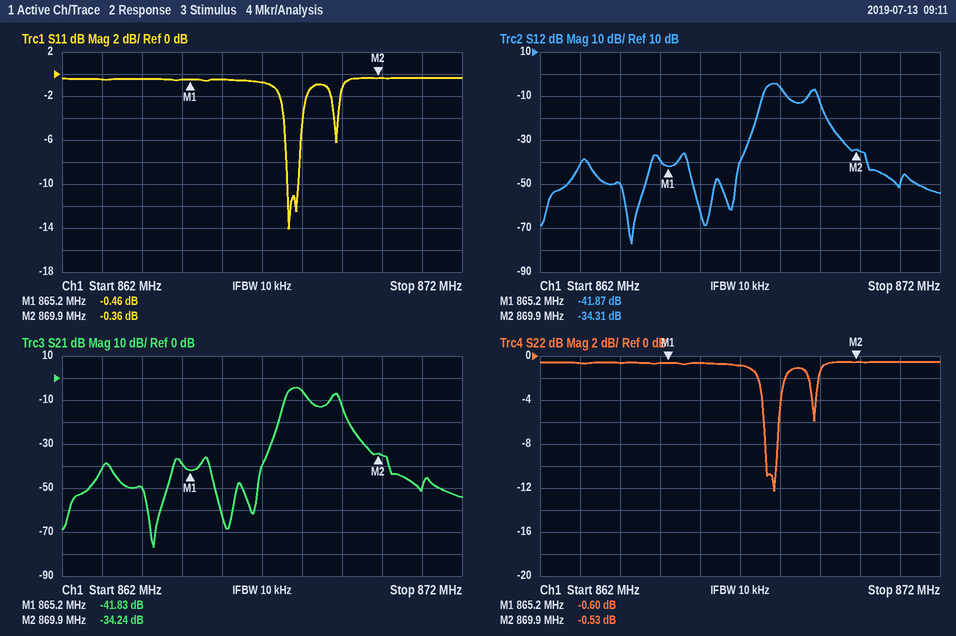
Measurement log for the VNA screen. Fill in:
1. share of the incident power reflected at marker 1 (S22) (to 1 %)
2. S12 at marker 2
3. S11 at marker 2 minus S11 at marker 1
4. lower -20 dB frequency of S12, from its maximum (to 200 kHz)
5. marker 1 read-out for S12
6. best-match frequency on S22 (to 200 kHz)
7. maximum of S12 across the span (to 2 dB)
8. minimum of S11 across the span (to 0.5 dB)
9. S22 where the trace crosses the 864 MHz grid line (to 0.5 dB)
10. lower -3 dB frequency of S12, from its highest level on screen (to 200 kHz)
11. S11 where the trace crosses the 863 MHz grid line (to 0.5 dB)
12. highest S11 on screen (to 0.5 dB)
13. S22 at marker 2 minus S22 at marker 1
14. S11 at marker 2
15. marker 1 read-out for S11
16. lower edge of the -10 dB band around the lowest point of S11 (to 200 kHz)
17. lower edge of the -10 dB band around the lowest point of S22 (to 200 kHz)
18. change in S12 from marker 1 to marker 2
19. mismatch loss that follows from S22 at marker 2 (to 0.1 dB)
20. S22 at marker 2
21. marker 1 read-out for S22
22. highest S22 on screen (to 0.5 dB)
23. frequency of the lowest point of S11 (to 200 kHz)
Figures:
87 %
-34.31 dB
0.10 dB
867.4 MHz
-41.87 dB
867.8 MHz
-4 dB
-14.0 dB
-0.5 dB
867.6 MHz
-0.5 dB
-0.5 dB
0.07 dB
-0.36 dB
-0.46 dB
867.6 MHz
867.6 MHz
7.56 dB
9.4 dB
-0.53 dB
-0.60 dB
-0.5 dB
867.6 MHz
